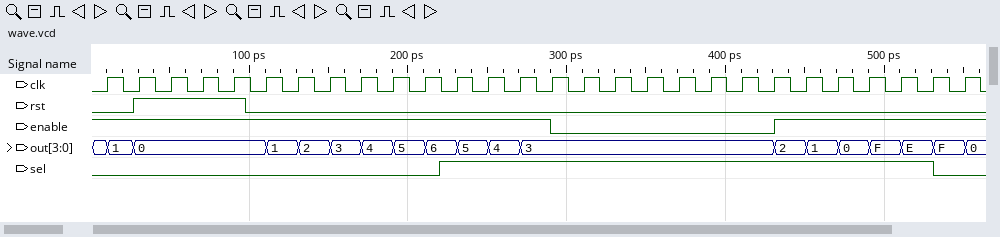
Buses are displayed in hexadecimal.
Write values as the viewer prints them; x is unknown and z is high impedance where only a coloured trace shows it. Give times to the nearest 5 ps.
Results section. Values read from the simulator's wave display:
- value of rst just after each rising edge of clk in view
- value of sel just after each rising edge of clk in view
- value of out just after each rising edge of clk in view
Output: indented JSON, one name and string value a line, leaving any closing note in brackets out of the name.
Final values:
{
  "value of rst just after each rising edge of clk in view": "0 1 1 1 1 0 0 0 0 0 0 0 0 0 0 0 0 0 0 0 0 0 0 0 0 0 0 0",
  "value of sel just after each rising edge of clk in view": "0 0 0 0 0 0 0 0 0 0 0 1 1 1 1 1 1 1 1 1 1 1 1 1 1 1 0 0",
  "value of out just after each rising edge of clk in view": "1, 0, 0, 0, 0, 1, 2, 3, 4, 5, 6, 5, 4, 3, 3, 3, 3, 3, 3, 3, 3, 2, 1, 0, F, E, F, 0"
}
